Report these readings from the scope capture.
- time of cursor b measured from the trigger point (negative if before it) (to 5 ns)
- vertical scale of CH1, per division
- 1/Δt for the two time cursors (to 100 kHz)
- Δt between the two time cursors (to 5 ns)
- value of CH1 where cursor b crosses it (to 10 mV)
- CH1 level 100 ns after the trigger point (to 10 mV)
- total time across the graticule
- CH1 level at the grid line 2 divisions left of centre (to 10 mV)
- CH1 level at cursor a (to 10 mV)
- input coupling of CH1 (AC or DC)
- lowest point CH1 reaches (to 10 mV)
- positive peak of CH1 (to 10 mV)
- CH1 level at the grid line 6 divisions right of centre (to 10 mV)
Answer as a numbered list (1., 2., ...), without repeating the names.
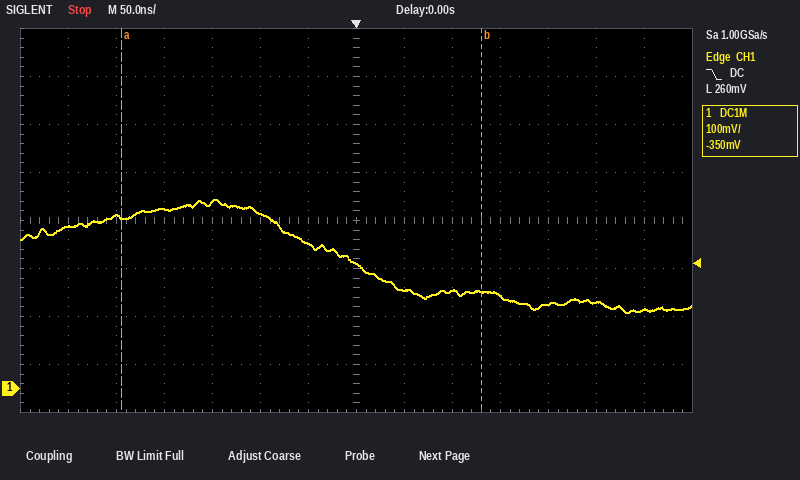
1. +130 ns
2. 100 mV
3. 2.7 MHz
4. 375 ns
5. 200 mV
6. 200 mV
7. 700 ns
8. 360 mV
9. 360 mV
10. DC
11. 160 mV
12. 390 mV
13. 160 mV
